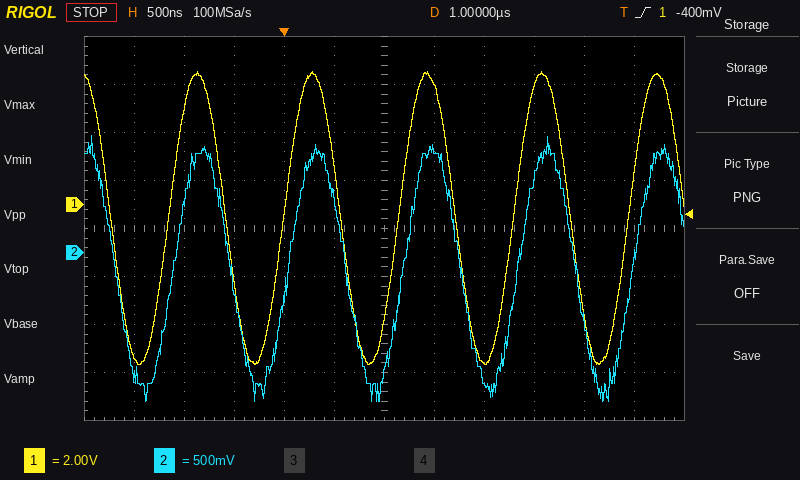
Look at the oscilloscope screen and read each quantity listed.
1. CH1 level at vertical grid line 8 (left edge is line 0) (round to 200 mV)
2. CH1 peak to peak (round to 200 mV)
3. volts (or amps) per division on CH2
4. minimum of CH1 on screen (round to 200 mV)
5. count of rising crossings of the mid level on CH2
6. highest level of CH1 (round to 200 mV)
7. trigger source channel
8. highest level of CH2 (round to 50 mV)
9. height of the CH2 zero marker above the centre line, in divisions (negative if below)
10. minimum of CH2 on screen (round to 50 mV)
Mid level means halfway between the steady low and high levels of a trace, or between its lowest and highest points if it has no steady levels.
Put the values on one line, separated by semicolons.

-6.6 V; 12.2 V; 500 mV; -6.6 V; 5; 5.6 V; CH1; 1.20 V; -0.5 div; -1.55 V
